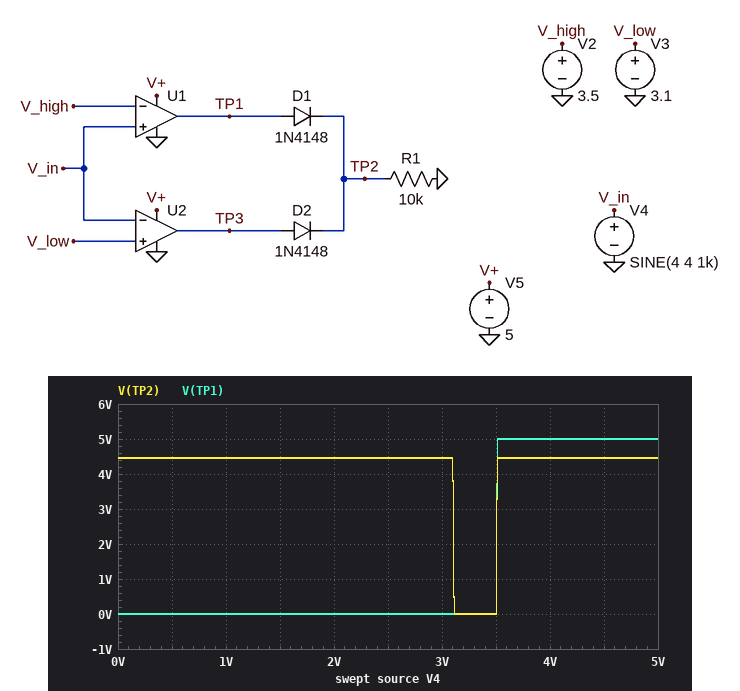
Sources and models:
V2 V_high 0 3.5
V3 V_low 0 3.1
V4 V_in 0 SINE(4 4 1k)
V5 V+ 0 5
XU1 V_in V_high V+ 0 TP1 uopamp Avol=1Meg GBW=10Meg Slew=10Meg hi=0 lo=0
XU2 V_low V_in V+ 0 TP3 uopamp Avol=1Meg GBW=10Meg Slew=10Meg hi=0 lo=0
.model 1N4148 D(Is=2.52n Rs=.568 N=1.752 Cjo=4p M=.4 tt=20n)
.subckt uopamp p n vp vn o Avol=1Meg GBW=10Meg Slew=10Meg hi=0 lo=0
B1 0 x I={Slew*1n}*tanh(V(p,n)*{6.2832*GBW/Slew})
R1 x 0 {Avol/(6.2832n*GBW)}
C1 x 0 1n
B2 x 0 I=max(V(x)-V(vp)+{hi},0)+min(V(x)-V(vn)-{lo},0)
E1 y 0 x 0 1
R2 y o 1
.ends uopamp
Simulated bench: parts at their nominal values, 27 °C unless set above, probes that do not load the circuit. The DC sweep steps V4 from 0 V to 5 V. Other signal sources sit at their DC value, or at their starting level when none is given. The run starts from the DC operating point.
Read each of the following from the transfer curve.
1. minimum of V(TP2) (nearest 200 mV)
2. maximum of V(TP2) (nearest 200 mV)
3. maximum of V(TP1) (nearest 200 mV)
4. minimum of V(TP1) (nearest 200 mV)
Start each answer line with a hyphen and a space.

- 0 V
- 4.4 V
- 5.0 V
- 0 V
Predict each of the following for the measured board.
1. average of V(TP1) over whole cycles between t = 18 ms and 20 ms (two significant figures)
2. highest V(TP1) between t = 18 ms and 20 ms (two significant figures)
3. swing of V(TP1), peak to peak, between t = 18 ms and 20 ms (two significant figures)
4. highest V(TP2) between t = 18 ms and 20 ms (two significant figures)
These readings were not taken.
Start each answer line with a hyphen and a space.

- 2.7 V
- 5.0 V
- 5.0 V
- 4.5 V
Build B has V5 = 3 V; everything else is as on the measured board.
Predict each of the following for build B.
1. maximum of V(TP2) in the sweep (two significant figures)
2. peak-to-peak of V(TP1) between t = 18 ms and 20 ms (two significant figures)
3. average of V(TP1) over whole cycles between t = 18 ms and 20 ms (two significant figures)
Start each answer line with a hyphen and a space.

- 2.5 V
- 3.0 V
- 1.6 V
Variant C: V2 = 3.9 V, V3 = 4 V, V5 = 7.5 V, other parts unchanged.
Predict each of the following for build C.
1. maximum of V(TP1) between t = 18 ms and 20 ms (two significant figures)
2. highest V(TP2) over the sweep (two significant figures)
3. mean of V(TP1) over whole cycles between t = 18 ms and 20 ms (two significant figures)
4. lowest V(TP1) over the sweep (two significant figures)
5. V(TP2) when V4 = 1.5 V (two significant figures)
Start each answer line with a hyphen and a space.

- 7.5 V
- 7.0 V
- 3.8 V
- -10 mV
- 6.9 V
